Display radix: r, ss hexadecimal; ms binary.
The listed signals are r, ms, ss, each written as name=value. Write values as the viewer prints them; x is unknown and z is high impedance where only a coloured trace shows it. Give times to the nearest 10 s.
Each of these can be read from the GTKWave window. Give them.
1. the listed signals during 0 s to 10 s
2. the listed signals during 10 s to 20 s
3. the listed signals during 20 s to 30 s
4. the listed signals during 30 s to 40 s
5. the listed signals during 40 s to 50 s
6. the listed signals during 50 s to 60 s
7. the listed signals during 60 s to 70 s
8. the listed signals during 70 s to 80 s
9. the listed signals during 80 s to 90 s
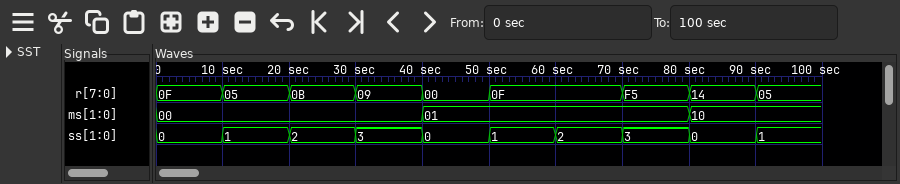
r=0F, ms=00, ss=0
r=05, ms=00, ss=1
r=0B, ms=00, ss=2
r=09, ms=00, ss=3
r=00, ms=01, ss=0
r=0F, ms=01, ss=1
r=0F, ms=01, ss=2
r=F5, ms=01, ss=3
r=14, ms=10, ss=0
